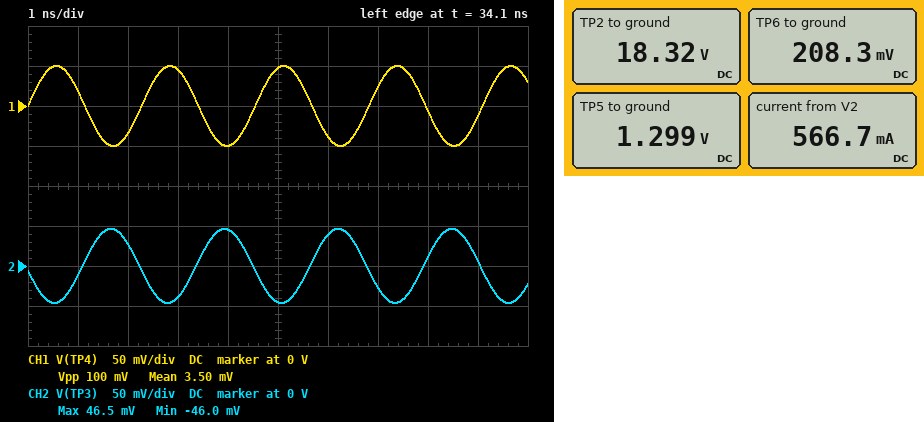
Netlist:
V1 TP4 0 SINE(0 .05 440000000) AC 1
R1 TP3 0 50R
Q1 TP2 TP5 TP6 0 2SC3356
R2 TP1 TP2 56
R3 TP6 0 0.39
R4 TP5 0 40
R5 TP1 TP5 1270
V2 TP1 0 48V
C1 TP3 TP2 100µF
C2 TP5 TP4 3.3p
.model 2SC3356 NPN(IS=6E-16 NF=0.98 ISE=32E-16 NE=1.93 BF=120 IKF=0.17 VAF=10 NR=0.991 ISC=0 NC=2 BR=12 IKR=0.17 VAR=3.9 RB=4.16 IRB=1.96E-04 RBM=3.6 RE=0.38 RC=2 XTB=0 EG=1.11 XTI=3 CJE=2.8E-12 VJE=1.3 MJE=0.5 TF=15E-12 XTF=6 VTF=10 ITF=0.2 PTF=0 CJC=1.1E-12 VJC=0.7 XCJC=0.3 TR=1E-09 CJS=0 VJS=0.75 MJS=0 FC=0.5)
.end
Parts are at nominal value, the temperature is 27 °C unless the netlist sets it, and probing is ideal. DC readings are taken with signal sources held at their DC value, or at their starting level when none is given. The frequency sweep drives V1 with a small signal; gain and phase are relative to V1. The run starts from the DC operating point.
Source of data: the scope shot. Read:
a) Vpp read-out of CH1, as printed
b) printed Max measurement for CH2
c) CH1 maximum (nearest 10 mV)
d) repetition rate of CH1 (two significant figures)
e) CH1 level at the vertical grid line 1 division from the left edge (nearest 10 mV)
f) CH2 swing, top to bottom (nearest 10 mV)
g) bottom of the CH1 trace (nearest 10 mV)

100 mV
46.5 mV
50 mV
440 MHz
20 mV
90 mV
-50 mV
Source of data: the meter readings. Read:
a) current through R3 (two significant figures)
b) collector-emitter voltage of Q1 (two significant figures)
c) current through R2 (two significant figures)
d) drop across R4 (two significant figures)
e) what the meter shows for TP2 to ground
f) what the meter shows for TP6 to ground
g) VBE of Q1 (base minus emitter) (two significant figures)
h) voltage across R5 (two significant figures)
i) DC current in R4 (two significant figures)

530 mA
18 V
530 mA
1.3 V
18.32 V
208.3 mV
1.1 V
47 V
32 mA
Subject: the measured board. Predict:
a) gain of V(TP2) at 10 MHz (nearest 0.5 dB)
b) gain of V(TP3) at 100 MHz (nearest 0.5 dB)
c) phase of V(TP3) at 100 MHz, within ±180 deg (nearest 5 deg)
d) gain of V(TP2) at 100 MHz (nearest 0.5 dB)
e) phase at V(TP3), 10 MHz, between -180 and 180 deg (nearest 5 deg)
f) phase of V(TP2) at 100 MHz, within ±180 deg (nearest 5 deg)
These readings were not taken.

-18.5 dB
-2.5 dB
-140 deg
-2.5 dB
-95 deg
-140 deg
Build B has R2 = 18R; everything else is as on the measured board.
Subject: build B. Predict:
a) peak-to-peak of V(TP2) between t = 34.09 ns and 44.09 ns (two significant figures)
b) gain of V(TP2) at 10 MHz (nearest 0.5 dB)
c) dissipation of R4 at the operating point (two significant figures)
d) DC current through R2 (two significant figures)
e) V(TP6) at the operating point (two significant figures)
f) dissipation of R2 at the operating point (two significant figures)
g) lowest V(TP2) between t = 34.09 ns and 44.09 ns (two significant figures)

120 mV
-20.5 dB
47 mW
650 mA
250 mV
7.6 W
36 V
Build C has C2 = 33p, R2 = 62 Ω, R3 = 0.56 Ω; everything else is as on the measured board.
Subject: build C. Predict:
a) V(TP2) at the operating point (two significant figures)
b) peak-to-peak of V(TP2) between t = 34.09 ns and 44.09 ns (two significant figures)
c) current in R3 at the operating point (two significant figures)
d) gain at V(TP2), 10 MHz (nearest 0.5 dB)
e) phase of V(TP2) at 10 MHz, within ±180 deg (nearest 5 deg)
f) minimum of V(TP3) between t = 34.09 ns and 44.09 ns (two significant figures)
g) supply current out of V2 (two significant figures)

19 V
750 mV
480 mA
1.5 dB
-100 deg
-370 mV
510 mA
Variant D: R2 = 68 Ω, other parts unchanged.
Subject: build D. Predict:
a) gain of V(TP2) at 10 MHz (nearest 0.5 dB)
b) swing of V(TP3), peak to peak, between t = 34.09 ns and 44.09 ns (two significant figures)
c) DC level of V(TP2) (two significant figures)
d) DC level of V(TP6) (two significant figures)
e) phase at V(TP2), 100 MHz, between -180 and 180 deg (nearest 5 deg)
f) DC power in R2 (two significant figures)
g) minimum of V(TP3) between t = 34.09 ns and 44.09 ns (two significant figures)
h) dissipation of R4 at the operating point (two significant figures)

-19.5 dB
80 mV
15 V
190 mV
-145 deg
16 W
-40 mV
41 mW
